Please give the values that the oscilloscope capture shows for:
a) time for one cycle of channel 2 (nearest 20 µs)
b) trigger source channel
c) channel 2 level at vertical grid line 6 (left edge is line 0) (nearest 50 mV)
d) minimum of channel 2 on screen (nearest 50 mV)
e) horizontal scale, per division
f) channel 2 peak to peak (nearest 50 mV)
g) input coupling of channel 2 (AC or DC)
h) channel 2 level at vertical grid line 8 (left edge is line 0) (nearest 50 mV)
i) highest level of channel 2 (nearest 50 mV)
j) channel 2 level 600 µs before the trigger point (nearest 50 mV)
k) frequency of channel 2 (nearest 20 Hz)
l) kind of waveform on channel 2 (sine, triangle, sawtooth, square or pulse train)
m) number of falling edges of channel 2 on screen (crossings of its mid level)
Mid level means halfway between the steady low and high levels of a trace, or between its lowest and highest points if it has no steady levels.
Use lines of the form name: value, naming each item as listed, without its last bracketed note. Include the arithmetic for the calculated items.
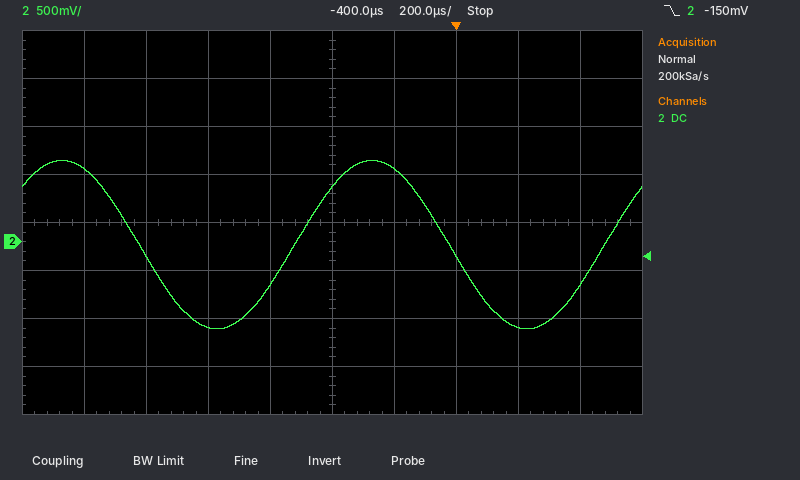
time for one cycle of channel 2: 1.00 ms
trigger source channel: channel 2
channel 2 level at vertical grid line 6 (left edge is line 0): 750 mV
minimum of channel 2 on screen: -900 mV
horizontal scale, per division: 200 µs
channel 2 peak to peak: 850 mV − (-900 mV) = 1.75 V
input coupling of channel 2: DC
channel 2 level at vertical grid line 8 (left edge is line 0): -900 mV
highest level of channel 2: 850 mV
channel 2 level 600 µs before the trigger point: -450 mV
frequency of channel 2: 1 / 1.00 ms ≈ 1.00 kHz
kind of waveform on channel 2: sine
number of falling edges of channel 2 on screen: 2
